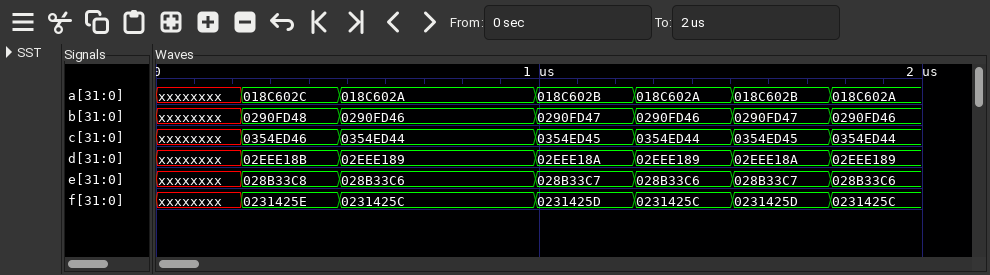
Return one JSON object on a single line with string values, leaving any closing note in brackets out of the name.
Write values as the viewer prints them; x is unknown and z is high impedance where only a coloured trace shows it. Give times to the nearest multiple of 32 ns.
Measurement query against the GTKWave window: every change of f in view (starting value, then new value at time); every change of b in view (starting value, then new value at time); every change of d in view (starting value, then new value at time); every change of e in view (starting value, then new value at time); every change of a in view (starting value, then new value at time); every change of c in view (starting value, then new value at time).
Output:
{"every change of f in view": "xxxxxxxx, 0231425E at 224 ns, 0231425C at 480 ns, 0231425D at 992 ns, 0231425C at 1248 ns, 0231425D at 1504 ns, 0231425C at 1760 ns", "every change of b in view": "xxxxxxxx, 0290FD48 at 224 ns, 0290FD46 at 480 ns, 0290FD47 at 992 ns, 0290FD46 at 1248 ns, 0290FD47 at 1504 ns, 0290FD46 at 1760 ns", "every change of d in view": "xxxxxxxx, 02EEE18B at 224 ns, 02EEE189 at 480 ns, 02EEE18A at 992 ns, 02EEE189 at 1248 ns, 02EEE18A at 1504 ns, 02EEE189 at 1760 ns", "every change of e in view": "xxxxxxxx, 028B33C8 at 224 ns, 028B33C6 at 480 ns, 028B33C7 at 992 ns, 028B33C6 at 1248 ns, 028B33C7 at 1504 ns, 028B33C6 at 1760 ns", "every change of a in view": "xxxxxxxx, 018C602C at 224 ns, 018C602A at 480 ns, 018C602B at 992 ns, 018C602A at 1248 ns, 018C602B at 1504 ns, 018C602A at 1760 ns", "every change of c in view": "xxxxxxxx, 0354ED46 at 224 ns, 0354ED44 at 480 ns, 0354ED45 at 992 ns, 0354ED44 at 1248 ns, 0354ED45 at 1504 ns, 0354ED44 at 1760 ns"}
